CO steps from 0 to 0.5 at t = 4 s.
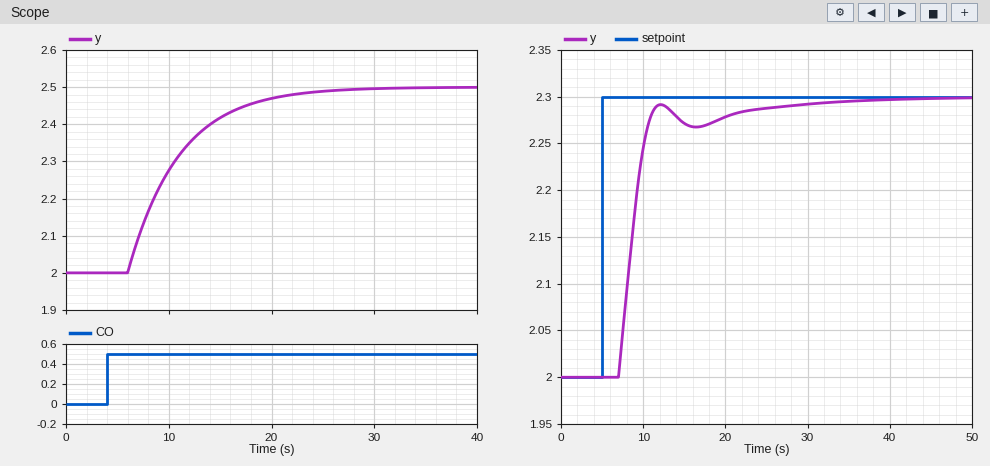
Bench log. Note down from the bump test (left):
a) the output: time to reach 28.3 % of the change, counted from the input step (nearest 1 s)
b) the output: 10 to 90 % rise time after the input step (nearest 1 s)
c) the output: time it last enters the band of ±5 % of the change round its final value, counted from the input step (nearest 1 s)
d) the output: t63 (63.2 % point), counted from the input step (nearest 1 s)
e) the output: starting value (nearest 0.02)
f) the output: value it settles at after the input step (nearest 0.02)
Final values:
4 s
11 s
17 s
7 s
2.00
2.50
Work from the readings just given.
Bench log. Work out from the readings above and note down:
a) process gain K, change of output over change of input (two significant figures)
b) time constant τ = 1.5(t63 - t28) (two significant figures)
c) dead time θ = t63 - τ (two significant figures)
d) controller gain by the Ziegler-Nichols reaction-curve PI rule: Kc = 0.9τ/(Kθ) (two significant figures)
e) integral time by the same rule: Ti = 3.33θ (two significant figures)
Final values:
1.0
4.5 s
2.5 s
1.6
8.3 s
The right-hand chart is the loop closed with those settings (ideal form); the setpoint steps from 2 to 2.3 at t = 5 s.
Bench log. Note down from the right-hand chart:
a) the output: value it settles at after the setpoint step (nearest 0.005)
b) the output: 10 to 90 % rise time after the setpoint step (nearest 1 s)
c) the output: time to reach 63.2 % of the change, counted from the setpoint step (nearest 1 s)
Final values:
2.300
3 s
4 s
